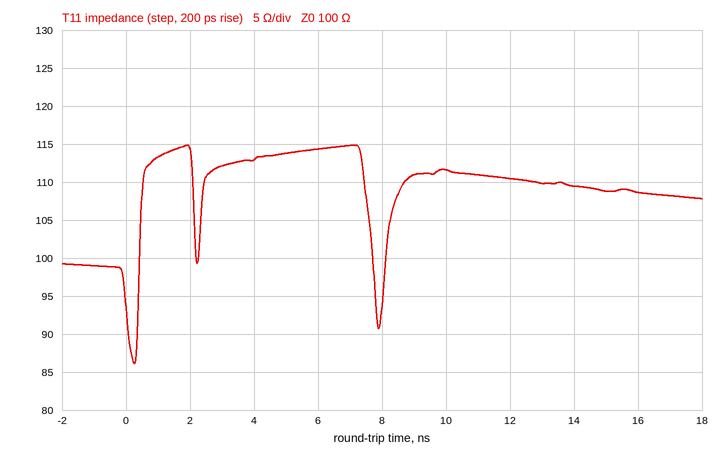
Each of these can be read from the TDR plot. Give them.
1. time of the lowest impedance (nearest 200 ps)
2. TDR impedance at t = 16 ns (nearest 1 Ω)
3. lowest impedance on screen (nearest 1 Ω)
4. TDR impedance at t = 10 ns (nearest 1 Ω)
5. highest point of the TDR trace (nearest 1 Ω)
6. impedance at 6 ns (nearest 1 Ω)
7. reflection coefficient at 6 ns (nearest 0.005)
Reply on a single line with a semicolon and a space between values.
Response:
200 ps; 109 Ω; 86 Ω; 112 Ω; 115 Ω; 114 Ω; +0.065
